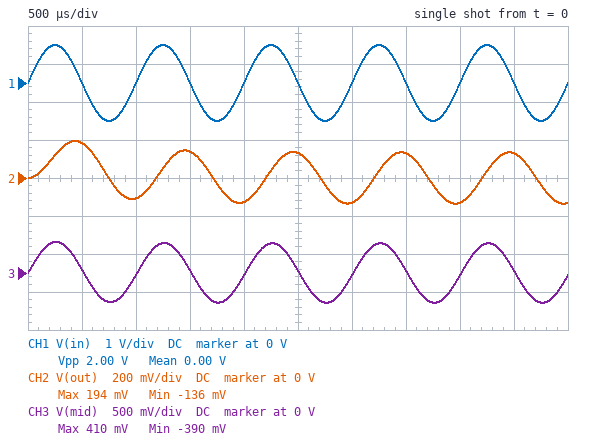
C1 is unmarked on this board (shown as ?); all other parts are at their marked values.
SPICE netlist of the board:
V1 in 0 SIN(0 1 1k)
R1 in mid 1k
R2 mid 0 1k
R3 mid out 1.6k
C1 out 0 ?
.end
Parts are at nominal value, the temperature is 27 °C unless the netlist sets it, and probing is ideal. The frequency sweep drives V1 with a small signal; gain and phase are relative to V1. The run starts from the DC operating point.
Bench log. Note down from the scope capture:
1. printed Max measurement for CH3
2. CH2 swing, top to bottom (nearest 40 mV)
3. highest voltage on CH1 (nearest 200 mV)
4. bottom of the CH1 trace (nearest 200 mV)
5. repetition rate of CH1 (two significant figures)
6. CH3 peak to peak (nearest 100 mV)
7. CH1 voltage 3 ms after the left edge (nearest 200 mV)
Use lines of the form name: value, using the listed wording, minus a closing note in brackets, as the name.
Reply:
printed Max measurement for CH3: 410 mV
CH2 swing, top to bottom: 320 mV
highest voltage on CH1: 1.0 V
bottom of the CH1 trace: -1.0 V
repetition rate of CH1: 1.0 kHz
CH3 peak to peak: 800 mV
CH1 voltage 3 ms after the left edge: 0 V
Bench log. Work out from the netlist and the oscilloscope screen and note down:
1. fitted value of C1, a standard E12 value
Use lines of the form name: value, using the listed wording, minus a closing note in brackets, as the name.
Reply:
fitted value of C1, a standard E12 value: 270 nF
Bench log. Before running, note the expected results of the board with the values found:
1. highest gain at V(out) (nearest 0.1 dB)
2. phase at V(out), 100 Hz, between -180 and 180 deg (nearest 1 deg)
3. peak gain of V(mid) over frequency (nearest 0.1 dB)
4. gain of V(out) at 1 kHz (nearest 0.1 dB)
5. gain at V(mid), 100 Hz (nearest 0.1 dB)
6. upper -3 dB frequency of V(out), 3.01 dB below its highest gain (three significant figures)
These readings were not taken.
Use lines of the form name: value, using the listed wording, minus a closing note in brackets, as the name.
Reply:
highest gain at V(out): -6.0 dB
phase at V(out), 100 Hz, between -180 and 180 deg: -20 deg
peak gain of V(mid) over frequency: -6.0 dB
gain of V(out) at 1 kHz: -17.4 dB
gain at V(mid), 100 Hz: -6.2 dB
upper -3 dB frequency of V(out), 3.01 dB below its highest gain: 281 Hz
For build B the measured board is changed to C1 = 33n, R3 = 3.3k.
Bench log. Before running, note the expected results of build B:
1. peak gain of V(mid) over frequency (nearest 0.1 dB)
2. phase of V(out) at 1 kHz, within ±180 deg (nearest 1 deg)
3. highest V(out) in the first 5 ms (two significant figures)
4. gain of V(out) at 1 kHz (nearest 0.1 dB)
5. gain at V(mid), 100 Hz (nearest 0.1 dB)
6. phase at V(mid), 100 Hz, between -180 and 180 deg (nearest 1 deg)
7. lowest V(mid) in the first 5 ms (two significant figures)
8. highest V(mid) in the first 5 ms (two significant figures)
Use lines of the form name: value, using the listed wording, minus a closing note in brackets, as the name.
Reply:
peak gain of V(mid) over frequency: -6.0 dB
phase of V(out) at 1 kHz, within ±180 deg: -38 deg
highest V(out) in the first 5 ms: 410 mV
gain of V(out) at 1 kHz: -8.1 dB
gain at V(mid), 100 Hz: -6.0 dB
phase at V(mid), 100 Hz, between -180 and 180 deg: -1 deg
lowest V(mid) in the first 5 ms: -480 mV
highest V(mid) in the first 5 ms: 480 mV
